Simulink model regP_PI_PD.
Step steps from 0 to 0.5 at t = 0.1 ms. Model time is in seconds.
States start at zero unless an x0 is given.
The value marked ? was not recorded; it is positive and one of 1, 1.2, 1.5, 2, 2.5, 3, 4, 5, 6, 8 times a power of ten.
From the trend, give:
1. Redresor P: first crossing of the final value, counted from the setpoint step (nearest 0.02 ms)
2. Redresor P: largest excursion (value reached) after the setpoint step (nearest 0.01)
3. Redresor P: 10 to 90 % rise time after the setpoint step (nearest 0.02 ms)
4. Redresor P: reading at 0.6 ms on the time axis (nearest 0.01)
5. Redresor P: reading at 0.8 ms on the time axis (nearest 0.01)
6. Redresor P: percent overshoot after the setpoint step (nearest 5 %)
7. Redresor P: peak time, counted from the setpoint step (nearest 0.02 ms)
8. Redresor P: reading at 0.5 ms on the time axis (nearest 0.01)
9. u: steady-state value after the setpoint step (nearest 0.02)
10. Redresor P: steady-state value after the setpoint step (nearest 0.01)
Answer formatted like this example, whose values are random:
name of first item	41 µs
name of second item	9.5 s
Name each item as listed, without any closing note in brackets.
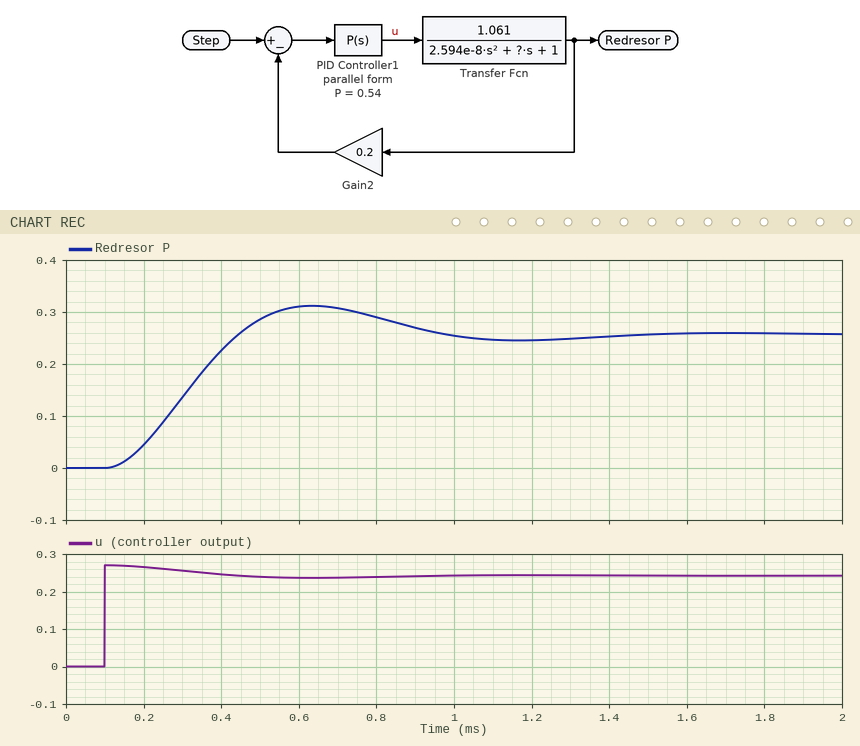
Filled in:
Redresor P: first crossing of the final value, counted from the setpoint step	0.34 ms
Redresor P: largest excursion (value reached) after the setpoint step	0.31
Redresor P: 10 to 90 % rise time after the setpoint step	0.24 ms
Redresor P: reading at 0.6 ms on the time axis	0.31
Redresor P: reading at 0.8 ms on the time axis	0.29
Redresor P: percent overshoot after the setpoint step	20 %
Redresor P: peak time, counted from the setpoint step	0.54 ms
Redresor P: reading at 0.5 ms on the time axis	0.29
u: steady-state value after the setpoint step	0.24
Redresor P: steady-state value after the setpoint step	0.26
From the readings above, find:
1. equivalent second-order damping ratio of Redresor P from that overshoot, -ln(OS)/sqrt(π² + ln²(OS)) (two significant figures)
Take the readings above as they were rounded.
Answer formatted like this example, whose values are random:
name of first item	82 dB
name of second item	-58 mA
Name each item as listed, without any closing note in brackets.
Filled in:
equivalent second-order damping ratio of Redresor P from that overshoot, -ln(OS)/sqrt(π² + ln²(OS))	0.46
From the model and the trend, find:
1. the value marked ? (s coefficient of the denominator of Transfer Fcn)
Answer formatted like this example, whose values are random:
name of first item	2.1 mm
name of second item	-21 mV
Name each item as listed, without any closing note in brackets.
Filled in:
the value marked ?	0.00015
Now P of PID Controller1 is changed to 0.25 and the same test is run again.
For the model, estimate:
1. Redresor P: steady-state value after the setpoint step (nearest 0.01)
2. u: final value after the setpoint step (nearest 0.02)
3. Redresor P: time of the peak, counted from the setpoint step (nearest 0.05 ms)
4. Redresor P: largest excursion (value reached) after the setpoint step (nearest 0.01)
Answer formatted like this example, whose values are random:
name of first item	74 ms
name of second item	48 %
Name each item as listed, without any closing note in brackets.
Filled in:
Redresor P: steady-state value after the setpoint step	0.13
u: final value after the setpoint step	0.12
Redresor P: time of the peak, counted from the setpoint step	0.55 ms
Redresor P: largest excursion (value reached) after the setpoint step	0.15
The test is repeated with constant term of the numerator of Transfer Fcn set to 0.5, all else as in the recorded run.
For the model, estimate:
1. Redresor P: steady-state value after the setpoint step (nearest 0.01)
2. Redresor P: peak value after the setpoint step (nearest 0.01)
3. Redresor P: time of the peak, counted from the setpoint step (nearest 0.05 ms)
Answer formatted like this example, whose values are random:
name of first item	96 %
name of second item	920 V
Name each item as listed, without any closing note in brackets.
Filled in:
Redresor P: steady-state value after the setpoint step	0.13
Redresor P: peak value after the setpoint step	0.15
Redresor P: time of the peak, counted from the setpoint step	0.55 ms
